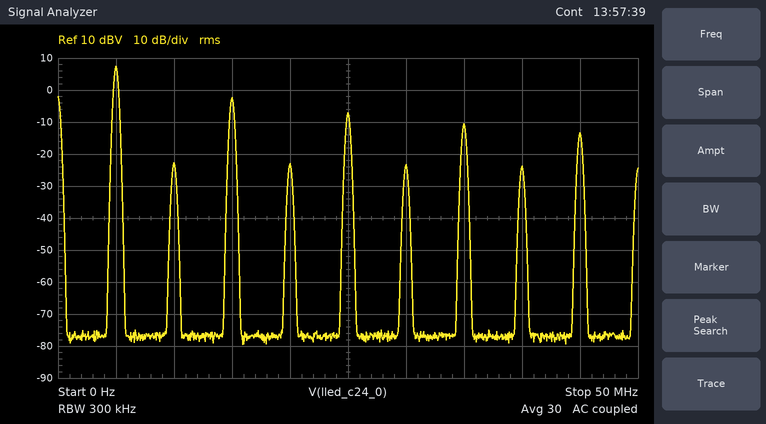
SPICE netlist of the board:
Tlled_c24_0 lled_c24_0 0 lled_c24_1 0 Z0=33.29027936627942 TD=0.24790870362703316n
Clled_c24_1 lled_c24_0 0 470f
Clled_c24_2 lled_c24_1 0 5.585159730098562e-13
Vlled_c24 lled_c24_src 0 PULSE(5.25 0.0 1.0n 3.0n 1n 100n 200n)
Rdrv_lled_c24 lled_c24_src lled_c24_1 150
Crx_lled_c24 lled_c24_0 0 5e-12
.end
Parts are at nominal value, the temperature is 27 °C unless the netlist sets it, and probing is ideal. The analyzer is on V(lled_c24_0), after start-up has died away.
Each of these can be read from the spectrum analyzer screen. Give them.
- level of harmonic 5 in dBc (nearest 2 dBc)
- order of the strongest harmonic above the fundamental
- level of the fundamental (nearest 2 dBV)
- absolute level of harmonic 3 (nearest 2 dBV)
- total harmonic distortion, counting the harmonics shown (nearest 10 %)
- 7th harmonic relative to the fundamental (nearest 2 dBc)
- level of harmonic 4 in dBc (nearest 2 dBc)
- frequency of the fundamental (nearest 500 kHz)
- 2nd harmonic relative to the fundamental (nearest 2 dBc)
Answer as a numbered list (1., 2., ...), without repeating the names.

1. -14 dBc
2. 3
3. 8 dBV
4. -2 dBV
5. 40 %
6. -18 dBc
7. -30 dBc
8. 5.0 MHz
9. -30 dBc
